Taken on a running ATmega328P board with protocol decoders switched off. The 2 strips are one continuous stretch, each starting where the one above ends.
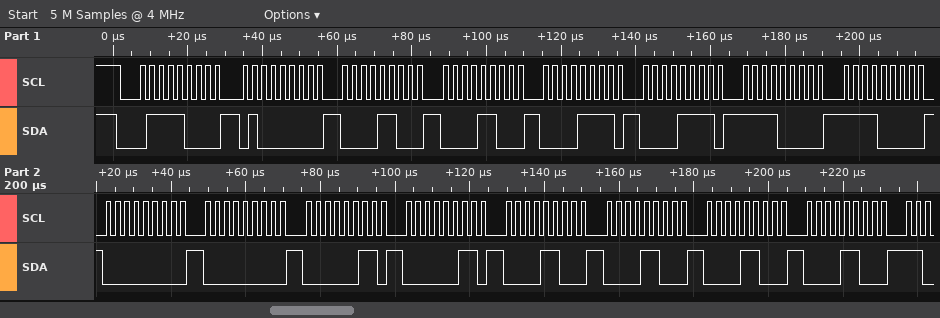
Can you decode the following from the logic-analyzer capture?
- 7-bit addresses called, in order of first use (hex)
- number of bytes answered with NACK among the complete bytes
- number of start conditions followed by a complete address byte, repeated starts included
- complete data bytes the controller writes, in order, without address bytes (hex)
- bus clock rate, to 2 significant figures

0x3C
0
1
40 0C 0C 0F 0F F0 F0 00 00 03 03 0C 0C 0C 0C
400 kHz
